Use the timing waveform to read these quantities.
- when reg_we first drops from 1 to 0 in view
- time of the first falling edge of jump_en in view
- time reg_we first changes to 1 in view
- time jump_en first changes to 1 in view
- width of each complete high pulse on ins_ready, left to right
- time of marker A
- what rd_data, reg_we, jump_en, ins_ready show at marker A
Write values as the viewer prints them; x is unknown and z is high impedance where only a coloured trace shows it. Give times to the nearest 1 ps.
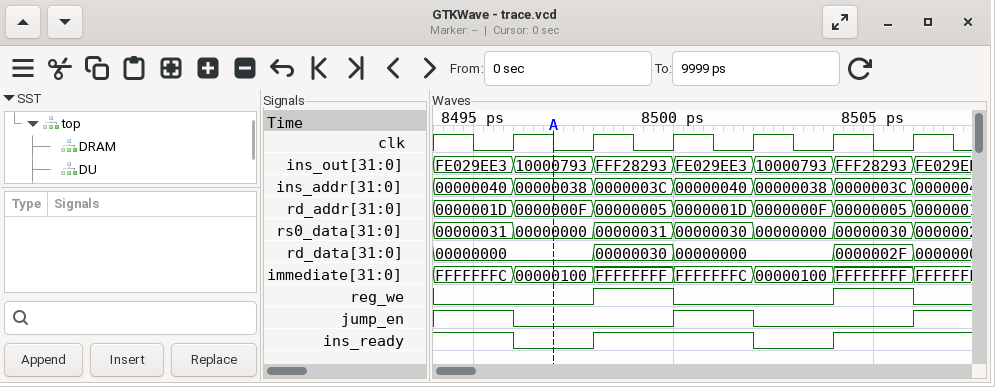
8500 ps
8496 ps
8498 ps
8500 ps
4 ps
8497 ps
rd_data=00000000, reg_we=0, jump_en=0, ins_ready=0
